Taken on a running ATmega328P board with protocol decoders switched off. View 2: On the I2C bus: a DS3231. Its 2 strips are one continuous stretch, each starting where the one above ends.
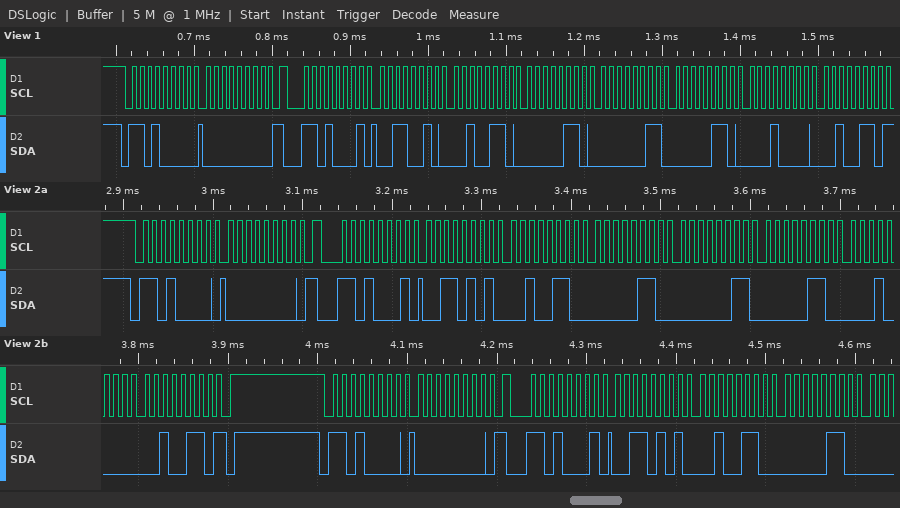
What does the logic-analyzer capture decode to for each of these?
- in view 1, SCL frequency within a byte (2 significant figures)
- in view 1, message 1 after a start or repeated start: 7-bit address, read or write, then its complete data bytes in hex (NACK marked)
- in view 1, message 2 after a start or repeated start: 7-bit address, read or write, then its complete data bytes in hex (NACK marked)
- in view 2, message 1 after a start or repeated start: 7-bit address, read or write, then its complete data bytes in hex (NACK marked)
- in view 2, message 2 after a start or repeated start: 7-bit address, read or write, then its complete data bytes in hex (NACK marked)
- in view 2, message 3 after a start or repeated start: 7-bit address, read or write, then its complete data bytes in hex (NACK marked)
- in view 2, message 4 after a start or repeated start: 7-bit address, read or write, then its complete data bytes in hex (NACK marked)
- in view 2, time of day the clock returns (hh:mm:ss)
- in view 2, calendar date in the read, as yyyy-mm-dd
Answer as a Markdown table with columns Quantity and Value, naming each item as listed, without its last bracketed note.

| Quantity | Value |
|---|---|
| in view 1, SCL frequency within a byte | 100 kHz |
| in view 1, message 1 after a start or repeated start: 7-bit address, read or write, then its complete data bytes in hex | 0x68 write: 00 |
| in view 1, message 2 after a start or repeated start: 7-bit address, read or write, then its complete data bytes in hex | 0x68 read: 32 26 06 03 06 10 26 NACK |
| in view 2, message 1 after a start or repeated start: 7-bit address, read or write, then its complete data bytes in hex | 0x68 write: 00 |
| in view 2, message 2 after a start or repeated start: 7-bit address, read or write, then its complete data bytes in hex | 0x68 read: 35 26 06 03 06 10 26 NACK |
| in view 2, message 3 after a start or repeated start: 7-bit address, read or write, then its complete data bytes in hex | 0x68 write: 00 |
| in view 2, message 4 after a start or repeated start: 7-bit address, read or write, then its complete data bytes in hex | 0x68 read: 35 26 06 |
| in view 2, time of day the clock returns | 06:26:35 |
| in view 2, calendar date in the read, as yyyy-mm-dd | 2026-10-06 |
